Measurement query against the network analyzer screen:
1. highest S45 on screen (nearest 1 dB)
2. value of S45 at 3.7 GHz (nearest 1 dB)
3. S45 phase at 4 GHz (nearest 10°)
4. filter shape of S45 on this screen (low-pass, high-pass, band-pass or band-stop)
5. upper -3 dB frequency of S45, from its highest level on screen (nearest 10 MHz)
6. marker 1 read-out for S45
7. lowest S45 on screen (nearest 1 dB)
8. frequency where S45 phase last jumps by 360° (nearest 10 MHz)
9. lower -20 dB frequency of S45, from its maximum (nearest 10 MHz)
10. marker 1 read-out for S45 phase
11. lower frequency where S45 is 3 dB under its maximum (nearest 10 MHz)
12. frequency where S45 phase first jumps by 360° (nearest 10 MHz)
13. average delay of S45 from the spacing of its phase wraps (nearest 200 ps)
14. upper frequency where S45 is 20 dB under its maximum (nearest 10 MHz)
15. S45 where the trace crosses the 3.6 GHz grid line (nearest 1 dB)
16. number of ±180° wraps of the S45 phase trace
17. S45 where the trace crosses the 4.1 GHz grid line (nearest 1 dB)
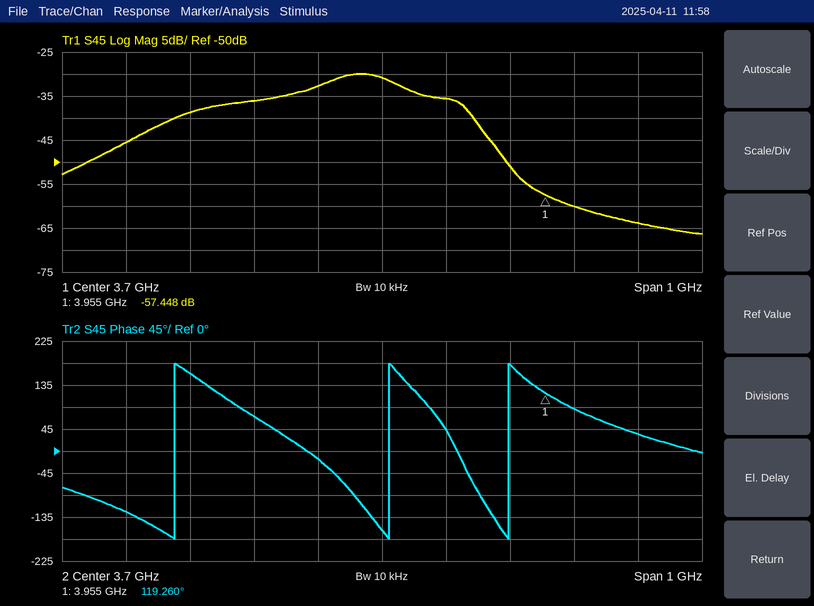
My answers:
-30 dB
-31 dB
90°
band-pass
3.73 GHz
-57.448 dB
-66 dB
3.90 GHz
3.24 GHz
119.260°
3.60 GHz
3.38 GHz
3.8 ns
3.89 GHz
-33 dB
3
-64 dB
